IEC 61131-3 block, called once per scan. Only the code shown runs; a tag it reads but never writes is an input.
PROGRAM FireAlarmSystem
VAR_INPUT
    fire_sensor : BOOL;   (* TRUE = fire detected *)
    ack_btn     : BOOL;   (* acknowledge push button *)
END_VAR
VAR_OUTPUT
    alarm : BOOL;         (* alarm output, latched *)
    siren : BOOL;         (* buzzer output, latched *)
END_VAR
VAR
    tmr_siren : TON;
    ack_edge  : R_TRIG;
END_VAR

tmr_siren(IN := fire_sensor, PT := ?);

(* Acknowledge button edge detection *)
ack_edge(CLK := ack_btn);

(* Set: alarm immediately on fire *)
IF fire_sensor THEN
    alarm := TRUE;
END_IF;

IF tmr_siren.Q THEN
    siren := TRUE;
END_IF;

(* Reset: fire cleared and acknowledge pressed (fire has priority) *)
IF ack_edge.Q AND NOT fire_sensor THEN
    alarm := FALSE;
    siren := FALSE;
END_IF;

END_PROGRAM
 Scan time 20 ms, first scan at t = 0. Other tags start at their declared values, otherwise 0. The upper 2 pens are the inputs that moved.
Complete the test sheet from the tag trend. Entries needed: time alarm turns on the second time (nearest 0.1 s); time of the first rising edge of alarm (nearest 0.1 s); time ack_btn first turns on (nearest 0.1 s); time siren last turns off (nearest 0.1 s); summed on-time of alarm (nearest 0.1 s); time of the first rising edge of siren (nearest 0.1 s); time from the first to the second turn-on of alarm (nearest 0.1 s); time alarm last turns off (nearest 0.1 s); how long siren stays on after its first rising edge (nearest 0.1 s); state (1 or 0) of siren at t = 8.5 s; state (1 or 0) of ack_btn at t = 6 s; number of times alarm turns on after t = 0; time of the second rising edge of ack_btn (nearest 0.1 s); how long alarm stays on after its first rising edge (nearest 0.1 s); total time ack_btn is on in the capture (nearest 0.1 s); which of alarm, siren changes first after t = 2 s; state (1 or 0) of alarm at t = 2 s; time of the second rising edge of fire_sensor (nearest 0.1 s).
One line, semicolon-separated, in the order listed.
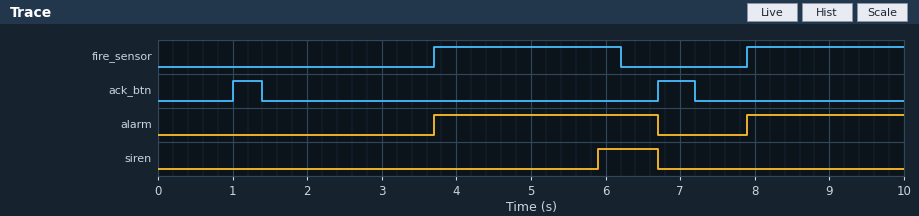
7.9 s; 3.7 s; 1.0 s; 6.7 s; 5.1 s; 5.9 s; 4.2 s; 6.7 s; 0.8 s; 0; 0; 2; 6.7 s; 3.0 s; 0.9 s; alarm; 0; 7.9 s
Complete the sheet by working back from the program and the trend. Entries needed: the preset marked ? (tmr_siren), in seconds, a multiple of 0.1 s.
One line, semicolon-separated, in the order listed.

2.2 s
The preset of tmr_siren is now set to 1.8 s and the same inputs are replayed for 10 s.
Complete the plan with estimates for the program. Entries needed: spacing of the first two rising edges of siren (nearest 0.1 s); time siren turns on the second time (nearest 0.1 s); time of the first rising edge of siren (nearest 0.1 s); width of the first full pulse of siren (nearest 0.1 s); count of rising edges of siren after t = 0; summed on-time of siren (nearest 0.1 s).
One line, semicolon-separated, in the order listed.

4.2 s; 9.7 s; 5.5 s; 1.2 s; 2; 1.5 s
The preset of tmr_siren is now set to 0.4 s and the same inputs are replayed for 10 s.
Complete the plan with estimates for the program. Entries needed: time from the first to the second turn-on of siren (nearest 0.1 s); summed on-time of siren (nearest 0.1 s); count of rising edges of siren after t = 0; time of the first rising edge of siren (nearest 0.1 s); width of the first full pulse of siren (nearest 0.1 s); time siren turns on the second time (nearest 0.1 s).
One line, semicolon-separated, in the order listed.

4.2 s; 4.3 s; 2; 4.1 s; 2.6 s; 8.3 s
